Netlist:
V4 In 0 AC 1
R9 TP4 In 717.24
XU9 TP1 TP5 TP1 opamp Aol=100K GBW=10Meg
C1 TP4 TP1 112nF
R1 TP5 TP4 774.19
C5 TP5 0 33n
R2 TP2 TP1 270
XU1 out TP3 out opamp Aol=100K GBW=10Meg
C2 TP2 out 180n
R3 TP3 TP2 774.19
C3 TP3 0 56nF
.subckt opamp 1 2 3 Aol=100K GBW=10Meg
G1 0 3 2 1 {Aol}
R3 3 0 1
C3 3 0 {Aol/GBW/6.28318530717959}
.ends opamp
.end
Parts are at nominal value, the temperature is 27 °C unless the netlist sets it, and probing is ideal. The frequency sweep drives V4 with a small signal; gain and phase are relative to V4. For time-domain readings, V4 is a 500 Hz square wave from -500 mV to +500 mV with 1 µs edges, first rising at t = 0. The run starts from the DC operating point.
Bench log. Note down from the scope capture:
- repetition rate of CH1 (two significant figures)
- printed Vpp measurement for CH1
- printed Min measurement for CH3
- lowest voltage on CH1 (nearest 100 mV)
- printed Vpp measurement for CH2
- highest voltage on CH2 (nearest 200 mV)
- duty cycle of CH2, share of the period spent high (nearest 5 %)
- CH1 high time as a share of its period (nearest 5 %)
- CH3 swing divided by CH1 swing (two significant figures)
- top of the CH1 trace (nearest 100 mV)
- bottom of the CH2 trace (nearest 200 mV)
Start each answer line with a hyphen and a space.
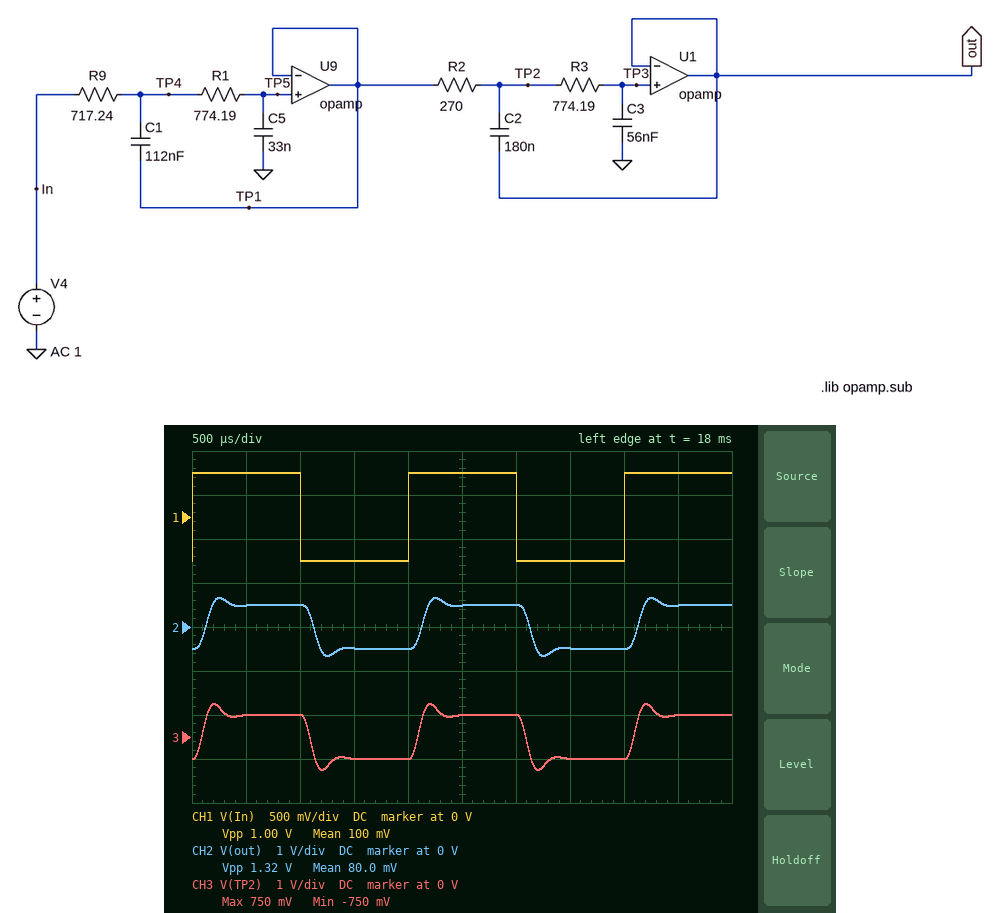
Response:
- 500 Hz
- 1.00 V
- -750 mV
- -500 mV
- 1.32 V
- 600 mV
- 50 %
- 50 %
- 1.5
- 500 mV
- -600 mV
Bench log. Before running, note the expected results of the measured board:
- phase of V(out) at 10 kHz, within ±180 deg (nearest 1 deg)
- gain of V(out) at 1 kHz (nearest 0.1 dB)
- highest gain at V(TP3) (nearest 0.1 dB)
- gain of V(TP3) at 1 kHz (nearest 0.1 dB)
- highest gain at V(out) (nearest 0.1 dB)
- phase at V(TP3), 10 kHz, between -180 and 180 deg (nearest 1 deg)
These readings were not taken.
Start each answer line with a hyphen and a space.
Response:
- 50 deg
- 0.4 dB
- 0.8 dB
- 0.4 dB
- 0.8 dB
- 50 deg
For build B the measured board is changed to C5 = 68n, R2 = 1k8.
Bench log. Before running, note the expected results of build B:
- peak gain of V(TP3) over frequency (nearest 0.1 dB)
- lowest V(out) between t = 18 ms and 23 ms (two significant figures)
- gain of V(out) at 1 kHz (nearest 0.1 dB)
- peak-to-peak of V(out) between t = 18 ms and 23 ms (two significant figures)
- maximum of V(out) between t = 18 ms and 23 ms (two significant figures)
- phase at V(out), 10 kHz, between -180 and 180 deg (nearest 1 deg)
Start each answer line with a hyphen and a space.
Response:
- 0.2 dB
- -590 mV
- -0.5 dB
- 1.2 V
- 590 mV
- 31 deg
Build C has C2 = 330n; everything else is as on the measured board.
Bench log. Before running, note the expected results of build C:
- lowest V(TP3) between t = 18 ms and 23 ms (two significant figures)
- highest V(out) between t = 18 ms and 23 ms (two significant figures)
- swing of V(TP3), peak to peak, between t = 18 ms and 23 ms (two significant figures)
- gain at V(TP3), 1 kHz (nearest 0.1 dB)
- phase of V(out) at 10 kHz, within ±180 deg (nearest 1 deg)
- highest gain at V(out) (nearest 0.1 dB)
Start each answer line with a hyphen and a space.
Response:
- -760 mV
- 760 mV
- 1.5 V
- 1.0 dB
- 38 deg
- 2.4 dB
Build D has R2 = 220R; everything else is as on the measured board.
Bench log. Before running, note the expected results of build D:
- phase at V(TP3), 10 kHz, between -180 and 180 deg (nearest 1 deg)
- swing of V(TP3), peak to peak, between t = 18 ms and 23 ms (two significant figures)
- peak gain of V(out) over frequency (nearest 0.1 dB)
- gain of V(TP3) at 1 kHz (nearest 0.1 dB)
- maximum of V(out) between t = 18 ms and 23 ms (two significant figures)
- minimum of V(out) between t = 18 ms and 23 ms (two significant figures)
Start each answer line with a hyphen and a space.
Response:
- 55 deg
- 1.3 V
- 0.7 dB
- 0.3 dB
- 650 mV
- -650 mV
